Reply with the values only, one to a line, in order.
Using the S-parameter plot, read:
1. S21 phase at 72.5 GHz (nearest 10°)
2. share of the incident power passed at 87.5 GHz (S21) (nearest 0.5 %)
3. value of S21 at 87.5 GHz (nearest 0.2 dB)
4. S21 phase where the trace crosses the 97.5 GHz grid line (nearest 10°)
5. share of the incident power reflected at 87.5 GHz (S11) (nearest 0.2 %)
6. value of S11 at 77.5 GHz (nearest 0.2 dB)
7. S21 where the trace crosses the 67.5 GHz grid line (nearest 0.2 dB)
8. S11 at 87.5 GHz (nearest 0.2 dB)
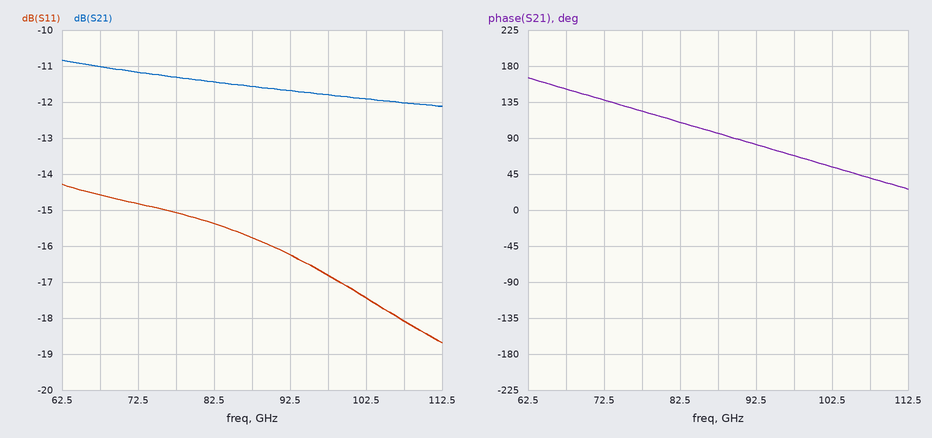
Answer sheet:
140°
7.0 %
-11.6 dB
70°
2.6 %
-15.0 dB
-11.0 dB
-15.8 dB
